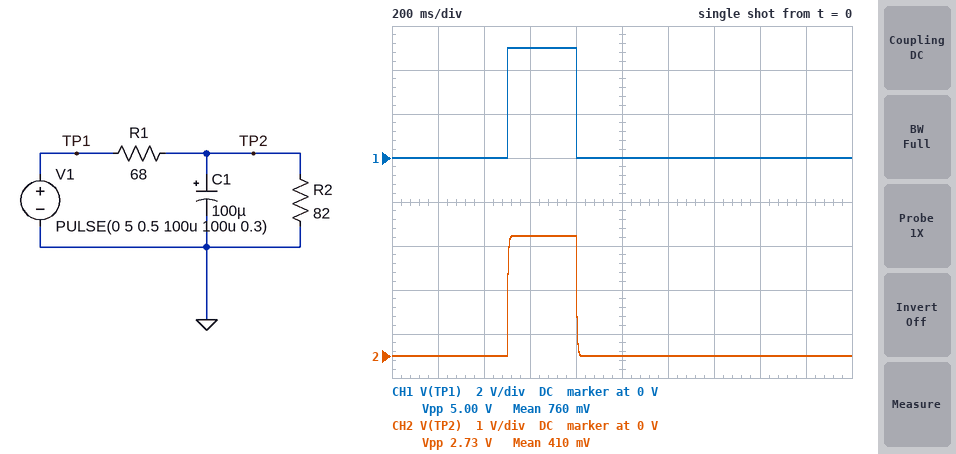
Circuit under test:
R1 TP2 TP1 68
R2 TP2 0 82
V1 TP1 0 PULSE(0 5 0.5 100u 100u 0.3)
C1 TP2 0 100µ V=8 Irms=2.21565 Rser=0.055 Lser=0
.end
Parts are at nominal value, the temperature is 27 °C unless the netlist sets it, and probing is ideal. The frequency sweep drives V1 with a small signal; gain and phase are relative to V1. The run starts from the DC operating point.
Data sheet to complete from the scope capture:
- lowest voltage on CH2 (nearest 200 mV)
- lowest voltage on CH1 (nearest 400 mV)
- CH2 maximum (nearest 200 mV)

0 V
0 V
2.8 V
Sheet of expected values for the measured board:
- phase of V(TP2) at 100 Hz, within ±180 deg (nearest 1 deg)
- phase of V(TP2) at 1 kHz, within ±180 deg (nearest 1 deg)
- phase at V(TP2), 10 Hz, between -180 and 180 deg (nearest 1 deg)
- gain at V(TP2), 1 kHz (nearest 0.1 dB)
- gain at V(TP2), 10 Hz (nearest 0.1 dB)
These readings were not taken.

-67 deg
-86 deg
-13 deg
-32.6 dB
-5.5 dB
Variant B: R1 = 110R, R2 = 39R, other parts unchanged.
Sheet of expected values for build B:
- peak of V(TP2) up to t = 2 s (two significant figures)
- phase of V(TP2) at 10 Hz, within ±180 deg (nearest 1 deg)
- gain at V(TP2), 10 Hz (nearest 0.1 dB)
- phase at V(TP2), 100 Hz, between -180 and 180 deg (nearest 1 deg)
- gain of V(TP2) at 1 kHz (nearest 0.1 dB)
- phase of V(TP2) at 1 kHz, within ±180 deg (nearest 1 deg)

1.3 V
-10 deg
-11.8 dB
-61 deg
-36.8 dB
-85 deg
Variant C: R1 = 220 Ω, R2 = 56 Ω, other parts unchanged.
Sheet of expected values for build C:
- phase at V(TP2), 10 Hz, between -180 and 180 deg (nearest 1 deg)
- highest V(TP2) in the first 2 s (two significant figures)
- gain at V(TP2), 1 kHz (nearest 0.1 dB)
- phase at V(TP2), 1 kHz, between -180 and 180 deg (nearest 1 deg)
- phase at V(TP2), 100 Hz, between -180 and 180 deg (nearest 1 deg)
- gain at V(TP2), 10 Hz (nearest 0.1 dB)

-16 deg
1.0 V
-42.8 dB
-86 deg
-70 deg
-14.2 dB
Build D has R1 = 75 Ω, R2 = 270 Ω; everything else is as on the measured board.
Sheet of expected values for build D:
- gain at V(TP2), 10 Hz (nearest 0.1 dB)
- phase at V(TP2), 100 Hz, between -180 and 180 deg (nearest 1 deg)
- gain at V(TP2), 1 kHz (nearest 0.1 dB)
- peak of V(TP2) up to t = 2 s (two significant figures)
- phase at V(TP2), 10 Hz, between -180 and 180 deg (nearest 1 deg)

-2.7 dB
-75 deg
-33.5 dB
3.9 V
-20 deg
